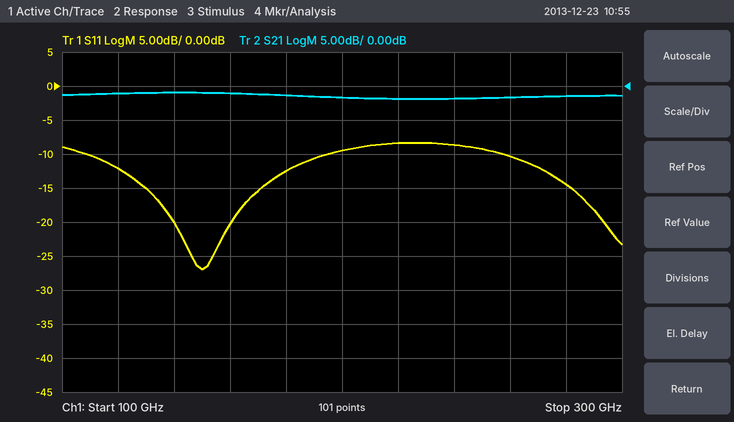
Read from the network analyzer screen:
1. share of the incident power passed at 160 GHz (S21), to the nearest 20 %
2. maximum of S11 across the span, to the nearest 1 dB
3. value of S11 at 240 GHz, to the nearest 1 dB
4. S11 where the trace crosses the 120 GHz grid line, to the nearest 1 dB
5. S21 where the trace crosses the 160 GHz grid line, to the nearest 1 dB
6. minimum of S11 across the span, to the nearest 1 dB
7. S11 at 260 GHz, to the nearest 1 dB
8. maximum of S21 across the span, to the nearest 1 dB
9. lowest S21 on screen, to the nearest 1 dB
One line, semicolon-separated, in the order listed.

80 %; -8 dB; -9 dB; -12 dB; -1 dB; -27 dB; -10 dB; -1 dB; -2 dB
